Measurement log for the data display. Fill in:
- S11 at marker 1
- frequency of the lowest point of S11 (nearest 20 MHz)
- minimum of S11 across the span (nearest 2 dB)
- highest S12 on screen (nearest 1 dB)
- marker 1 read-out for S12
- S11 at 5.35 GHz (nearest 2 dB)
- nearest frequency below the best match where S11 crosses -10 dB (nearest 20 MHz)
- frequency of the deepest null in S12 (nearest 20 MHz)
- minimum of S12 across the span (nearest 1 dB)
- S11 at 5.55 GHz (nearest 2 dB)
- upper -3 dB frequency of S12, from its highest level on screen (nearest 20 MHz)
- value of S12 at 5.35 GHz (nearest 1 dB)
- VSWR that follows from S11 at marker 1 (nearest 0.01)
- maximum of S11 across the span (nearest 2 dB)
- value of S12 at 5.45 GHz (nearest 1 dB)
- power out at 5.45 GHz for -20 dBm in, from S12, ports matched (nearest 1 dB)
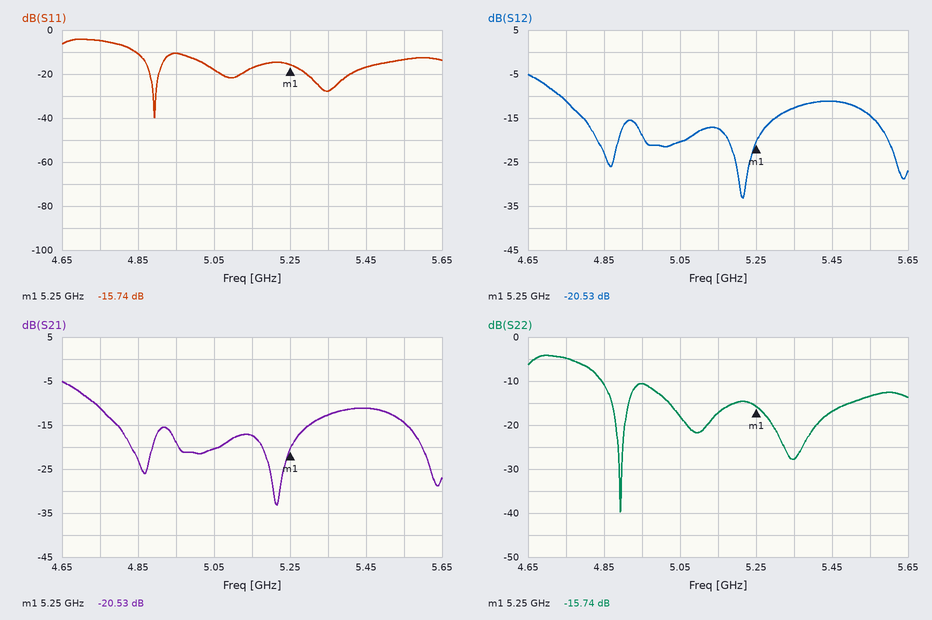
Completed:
-15.74 dB
4.90 GHz
-40 dB
-5 dB
-20.53 dB
-28 dB
4.84 GHz
5.22 GHz
-33 dB
-14 dB
4.70 GHz
-13 dB
1.39
-4 dB
-11 dB
-31 dBm
